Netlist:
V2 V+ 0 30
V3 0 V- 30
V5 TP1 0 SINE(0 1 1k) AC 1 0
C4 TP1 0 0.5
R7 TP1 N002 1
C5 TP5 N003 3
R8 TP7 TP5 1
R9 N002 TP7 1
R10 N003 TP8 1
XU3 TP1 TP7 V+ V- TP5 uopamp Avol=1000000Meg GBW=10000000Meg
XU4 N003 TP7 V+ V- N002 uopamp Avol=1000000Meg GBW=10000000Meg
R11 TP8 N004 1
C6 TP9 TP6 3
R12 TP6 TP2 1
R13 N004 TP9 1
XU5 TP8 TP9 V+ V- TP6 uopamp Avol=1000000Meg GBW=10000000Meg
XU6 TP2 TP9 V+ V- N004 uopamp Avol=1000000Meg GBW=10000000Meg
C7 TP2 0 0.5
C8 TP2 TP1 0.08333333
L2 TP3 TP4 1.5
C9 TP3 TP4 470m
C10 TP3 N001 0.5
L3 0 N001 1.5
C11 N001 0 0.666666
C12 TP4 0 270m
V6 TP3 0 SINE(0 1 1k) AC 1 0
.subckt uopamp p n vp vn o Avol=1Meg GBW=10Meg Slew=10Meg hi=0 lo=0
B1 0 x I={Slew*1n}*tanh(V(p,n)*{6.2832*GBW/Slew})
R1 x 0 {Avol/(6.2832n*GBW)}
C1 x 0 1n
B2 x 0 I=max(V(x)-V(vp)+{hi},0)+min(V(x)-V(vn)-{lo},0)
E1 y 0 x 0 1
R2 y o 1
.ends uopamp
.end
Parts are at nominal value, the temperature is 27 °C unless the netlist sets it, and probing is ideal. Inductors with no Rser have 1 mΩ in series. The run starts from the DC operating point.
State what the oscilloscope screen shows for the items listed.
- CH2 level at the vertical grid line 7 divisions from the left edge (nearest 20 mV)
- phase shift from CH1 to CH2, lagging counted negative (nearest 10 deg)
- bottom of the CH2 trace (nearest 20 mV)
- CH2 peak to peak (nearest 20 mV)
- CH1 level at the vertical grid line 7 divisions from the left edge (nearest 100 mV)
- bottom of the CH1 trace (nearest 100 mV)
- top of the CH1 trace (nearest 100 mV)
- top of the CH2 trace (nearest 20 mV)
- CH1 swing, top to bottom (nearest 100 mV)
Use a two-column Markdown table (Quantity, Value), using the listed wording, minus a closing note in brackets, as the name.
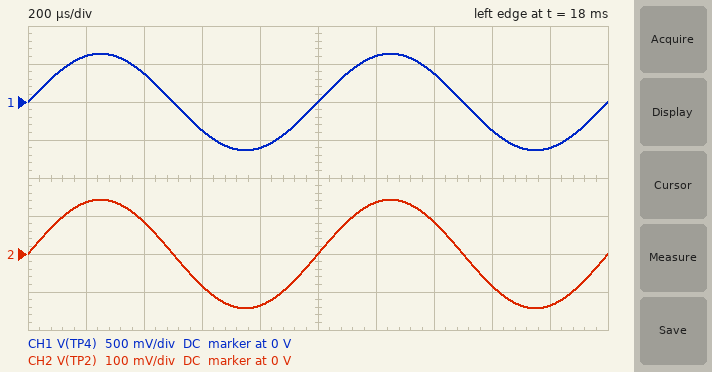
| Quantity | Value |
|---|---|
| CH2 level at the vertical grid line 7 divisions from the left edge | 80 mV |
| phase shift from CH1 to CH2, lagging counted negative | 0 deg |
| bottom of the CH2 trace | -140 mV |
| CH2 peak to peak | 280 mV |
| CH1 level at the vertical grid line 7 divisions from the left edge | 400 mV |
| bottom of the CH1 trace | -600 mV |
| top of the CH1 trace | 600 mV |
| top of the CH2 trace | 140 mV |
| CH1 swing, top to bottom | 1.3 V |
